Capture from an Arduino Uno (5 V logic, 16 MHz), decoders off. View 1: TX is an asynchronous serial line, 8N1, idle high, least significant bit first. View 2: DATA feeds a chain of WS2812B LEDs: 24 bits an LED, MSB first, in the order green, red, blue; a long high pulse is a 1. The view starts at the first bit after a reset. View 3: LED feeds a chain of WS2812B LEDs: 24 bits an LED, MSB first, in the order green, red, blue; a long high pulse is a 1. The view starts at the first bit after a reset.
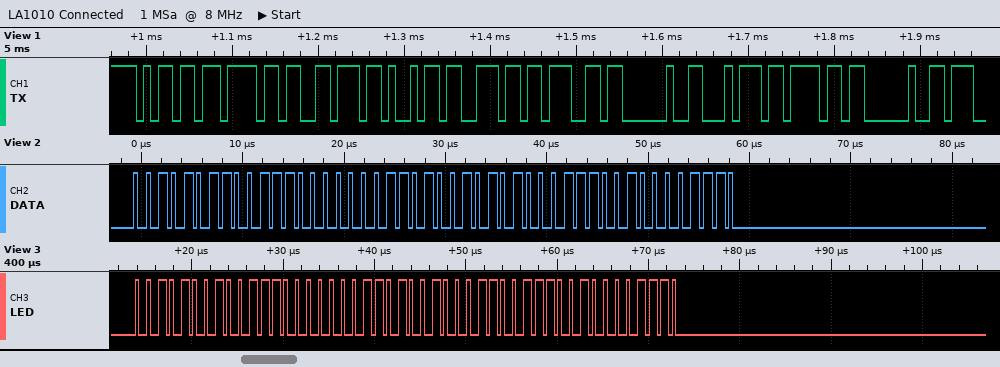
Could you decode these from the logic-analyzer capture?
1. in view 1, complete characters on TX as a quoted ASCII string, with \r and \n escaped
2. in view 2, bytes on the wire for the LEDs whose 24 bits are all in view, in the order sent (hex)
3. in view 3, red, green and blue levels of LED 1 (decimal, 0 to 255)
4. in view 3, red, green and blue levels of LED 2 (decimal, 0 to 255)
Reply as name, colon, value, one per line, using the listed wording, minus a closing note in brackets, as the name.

in view 1, complete characters on TX as a quoted ASCII string, with \r and \n escaped: "moving to "
in view 2, bytes on the wire for the LEDs whose 24 bits are all in view, in the order sent: 2B 38 0D 2A 39 0E
in view 3, red, green and blue levels of LED 1: 56, 41, 13
in view 3, red, green and blue levels of LED 2: 57, 35, 14
